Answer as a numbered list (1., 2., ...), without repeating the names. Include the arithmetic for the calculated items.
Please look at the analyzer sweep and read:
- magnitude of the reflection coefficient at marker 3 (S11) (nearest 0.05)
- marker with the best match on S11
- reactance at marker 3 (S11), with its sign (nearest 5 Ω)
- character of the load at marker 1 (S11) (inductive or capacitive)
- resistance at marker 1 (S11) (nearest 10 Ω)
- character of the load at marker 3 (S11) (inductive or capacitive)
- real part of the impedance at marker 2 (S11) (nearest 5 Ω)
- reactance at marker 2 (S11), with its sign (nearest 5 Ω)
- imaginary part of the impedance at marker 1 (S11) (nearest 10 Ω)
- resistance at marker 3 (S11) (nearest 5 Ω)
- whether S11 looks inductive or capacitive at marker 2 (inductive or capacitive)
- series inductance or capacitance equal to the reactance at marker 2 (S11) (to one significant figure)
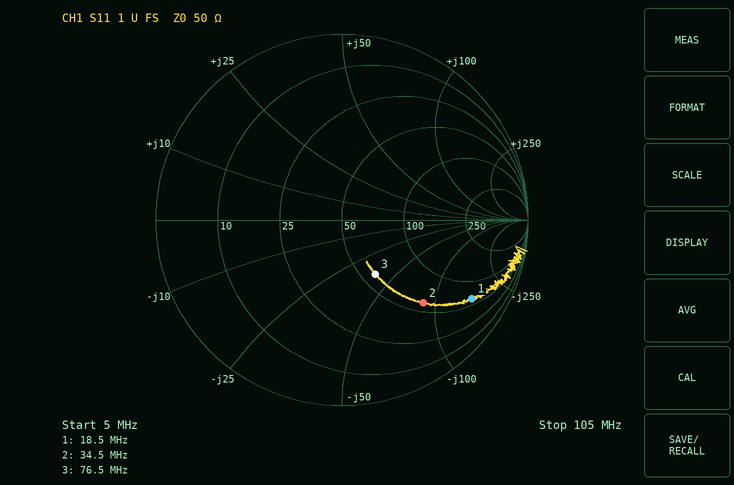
1. 0.35
2. marker 3
3. -40 Ω
4. capacitive
5. 60 Ω
6. capacitive
7. 60 Ω
8. -85 Ω
9. -160 Ω
10. 60 Ω
11. capacitive
12. C = 1/(2π × 34.5 MHz × 85 Ω) ≈ 54.3 pF, so 50 pF to one significant figure
